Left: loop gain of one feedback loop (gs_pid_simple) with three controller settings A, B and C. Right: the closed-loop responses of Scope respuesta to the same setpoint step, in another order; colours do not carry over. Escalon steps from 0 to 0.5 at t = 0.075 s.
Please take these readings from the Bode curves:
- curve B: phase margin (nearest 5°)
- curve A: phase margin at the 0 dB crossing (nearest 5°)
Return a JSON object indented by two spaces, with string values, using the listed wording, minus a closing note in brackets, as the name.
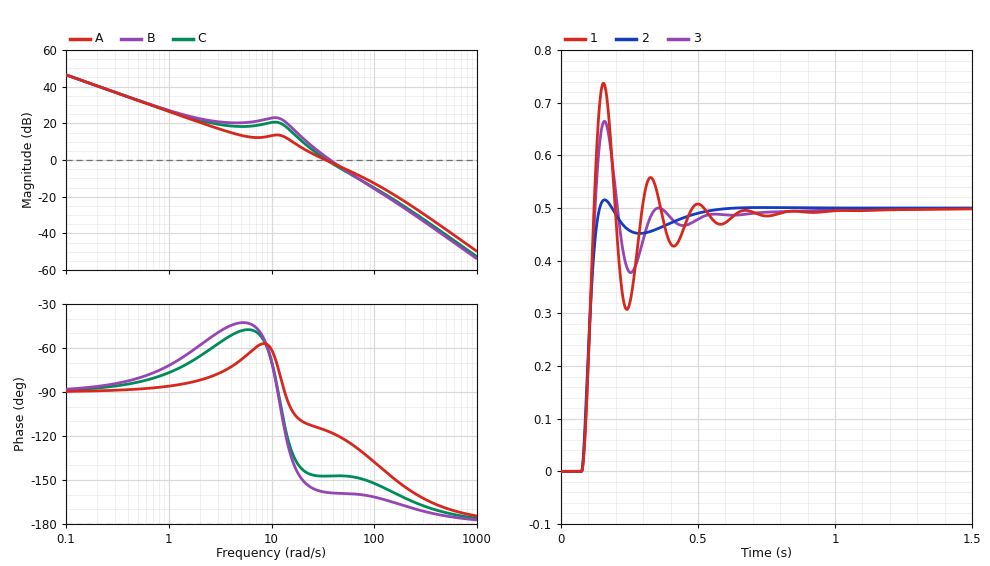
{
  "curve B: phase margin": "20°",
  "curve A: phase margin at the 0 dB crossing": "65°"
}
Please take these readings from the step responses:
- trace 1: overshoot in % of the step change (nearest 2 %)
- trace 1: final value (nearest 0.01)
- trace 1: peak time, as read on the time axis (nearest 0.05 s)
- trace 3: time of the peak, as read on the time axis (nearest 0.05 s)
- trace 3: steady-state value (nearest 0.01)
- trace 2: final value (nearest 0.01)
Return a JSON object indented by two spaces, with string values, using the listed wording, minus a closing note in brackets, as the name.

{
  "trace 1: overshoot in % of the step change": "48 %",
  "trace 1: final value": "0.50",
  "trace 1: peak time, as read on the time axis": "0.15 s",
  "trace 3: time of the peak, as read on the time axis": "0.15 s",
  "trace 3: steady-state value": "0.50",
  "trace 2: final value": "0.50"
}
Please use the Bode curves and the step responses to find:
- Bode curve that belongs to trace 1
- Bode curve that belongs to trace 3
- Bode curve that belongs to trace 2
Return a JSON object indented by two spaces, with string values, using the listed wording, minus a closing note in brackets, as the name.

{
  "Bode curve that belongs to trace 1": "B",
  "Bode curve that belongs to trace 3": "C",
  "Bode curve that belongs to trace 2": "A"
}
